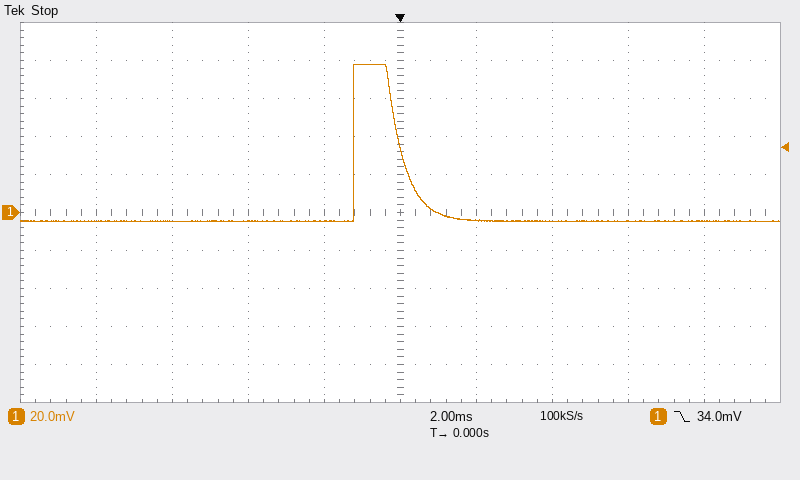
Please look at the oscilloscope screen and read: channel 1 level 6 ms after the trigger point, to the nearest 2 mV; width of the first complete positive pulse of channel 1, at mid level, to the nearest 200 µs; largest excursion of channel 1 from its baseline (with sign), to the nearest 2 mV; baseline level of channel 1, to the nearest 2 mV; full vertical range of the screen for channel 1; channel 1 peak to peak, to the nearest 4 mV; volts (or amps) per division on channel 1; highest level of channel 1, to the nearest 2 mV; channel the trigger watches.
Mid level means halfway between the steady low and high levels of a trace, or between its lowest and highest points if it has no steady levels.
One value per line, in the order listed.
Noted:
-4 mV
1.2 ms
+82 mV
-4 mV
200 mV
84 mV
20 mV
78 mV
channel 1
